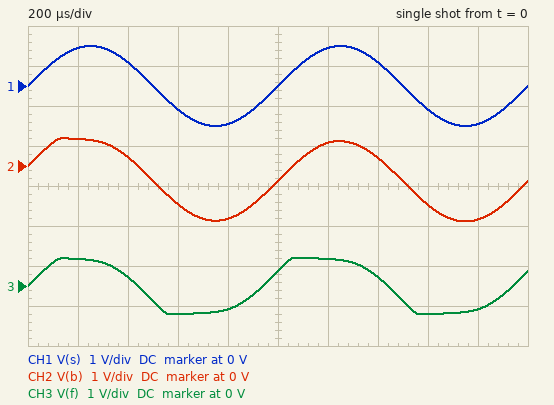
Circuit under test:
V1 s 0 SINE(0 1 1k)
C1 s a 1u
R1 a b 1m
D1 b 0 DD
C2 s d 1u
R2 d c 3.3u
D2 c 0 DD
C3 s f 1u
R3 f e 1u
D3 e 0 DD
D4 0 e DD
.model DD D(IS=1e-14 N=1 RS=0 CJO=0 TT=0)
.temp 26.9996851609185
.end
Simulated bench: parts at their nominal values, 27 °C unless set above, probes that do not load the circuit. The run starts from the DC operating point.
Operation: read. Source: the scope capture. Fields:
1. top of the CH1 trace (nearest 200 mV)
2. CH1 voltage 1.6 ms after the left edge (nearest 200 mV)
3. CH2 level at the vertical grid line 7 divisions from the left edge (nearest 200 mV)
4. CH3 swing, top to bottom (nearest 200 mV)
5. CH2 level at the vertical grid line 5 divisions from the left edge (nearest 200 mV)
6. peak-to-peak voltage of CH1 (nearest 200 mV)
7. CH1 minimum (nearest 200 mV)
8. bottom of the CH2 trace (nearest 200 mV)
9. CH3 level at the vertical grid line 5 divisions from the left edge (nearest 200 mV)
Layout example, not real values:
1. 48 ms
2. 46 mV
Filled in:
1. 1.0 V
2. -600 mV
3. 200 mV
4. 1.4 V
5. -400 mV
6. 2.0 V
7. -1.0 V
8. -1.4 V
9. 400 mV
